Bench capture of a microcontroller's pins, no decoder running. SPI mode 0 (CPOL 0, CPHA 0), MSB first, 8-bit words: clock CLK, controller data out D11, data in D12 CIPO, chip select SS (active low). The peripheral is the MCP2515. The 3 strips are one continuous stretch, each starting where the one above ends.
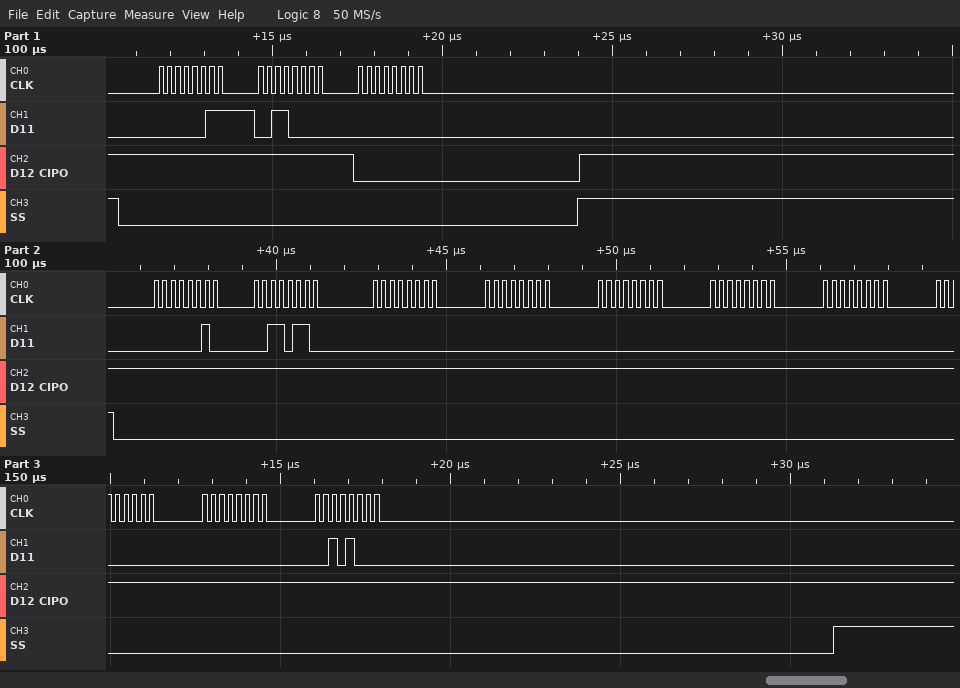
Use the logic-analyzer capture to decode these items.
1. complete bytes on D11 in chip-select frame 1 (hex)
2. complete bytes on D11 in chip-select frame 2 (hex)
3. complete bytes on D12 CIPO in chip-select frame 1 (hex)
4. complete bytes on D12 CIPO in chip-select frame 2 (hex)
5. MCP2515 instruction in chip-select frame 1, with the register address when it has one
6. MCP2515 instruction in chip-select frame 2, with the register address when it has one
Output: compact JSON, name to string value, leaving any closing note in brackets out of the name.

{"complete bytes on D11 in chip-select frame 1": "03 30 00", "complete bytes on D11 in chip-select frame 2": "02 36 00 00 00 00 00 00 00 28", "complete bytes on D12 CIPO in chip-select frame 1": "FF FF 00", "complete bytes on D12 CIPO in chip-select frame 2": "FF FF FF FF FF FF FF FF FF FF", "MCP2515 instruction in chip-select frame 1, with the register address when it has one": "READ 0x30", "MCP2515 instruction in chip-select frame 2, with the register address when it has one": "WRITE 0x36"}
